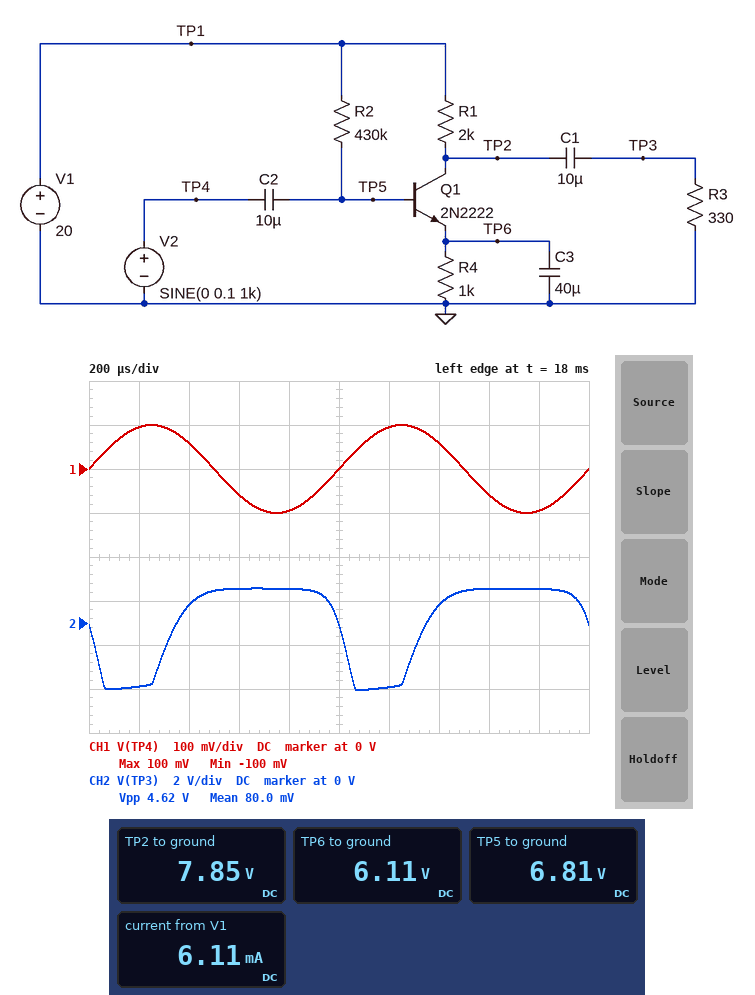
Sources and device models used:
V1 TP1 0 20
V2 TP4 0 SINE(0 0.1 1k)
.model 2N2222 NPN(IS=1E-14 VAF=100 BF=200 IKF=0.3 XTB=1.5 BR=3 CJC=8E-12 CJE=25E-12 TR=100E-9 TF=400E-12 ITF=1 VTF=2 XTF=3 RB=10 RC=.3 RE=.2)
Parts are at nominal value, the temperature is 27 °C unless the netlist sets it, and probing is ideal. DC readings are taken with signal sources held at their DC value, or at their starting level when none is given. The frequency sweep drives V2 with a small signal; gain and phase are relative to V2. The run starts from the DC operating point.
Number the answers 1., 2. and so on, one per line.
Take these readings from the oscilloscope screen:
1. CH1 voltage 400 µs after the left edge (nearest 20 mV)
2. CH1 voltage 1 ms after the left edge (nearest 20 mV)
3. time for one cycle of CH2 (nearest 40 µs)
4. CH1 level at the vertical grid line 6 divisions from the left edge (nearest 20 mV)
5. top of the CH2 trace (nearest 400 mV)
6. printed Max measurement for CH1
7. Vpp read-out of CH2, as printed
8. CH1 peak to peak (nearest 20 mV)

1. 60 mV
2. 0 V
3. 1.00 ms
4. 100 mV
5. 1.6 V
6. 100 mV
7. 4.62 V
8. 200 mV
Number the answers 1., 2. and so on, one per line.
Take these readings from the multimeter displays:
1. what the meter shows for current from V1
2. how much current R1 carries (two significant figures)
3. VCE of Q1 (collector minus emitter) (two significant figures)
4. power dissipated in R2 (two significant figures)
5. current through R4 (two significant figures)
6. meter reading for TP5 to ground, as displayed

1. 6.11 mA
2. 6.1 mA
3. 1.7 V
4. 400 µW
5. 6.1 mA
6. 6.81 V
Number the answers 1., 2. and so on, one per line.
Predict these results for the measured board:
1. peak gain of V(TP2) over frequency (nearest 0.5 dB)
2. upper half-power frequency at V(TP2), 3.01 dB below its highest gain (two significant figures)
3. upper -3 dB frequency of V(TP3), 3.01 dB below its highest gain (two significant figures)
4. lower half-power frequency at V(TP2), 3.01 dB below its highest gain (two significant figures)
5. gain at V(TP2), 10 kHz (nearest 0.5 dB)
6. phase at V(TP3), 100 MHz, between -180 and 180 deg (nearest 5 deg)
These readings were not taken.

1. 35.5 dB
2. 25 MHz
3. 25 MHz
4. 880 Hz
5. 35.5 dB
6. 90 deg
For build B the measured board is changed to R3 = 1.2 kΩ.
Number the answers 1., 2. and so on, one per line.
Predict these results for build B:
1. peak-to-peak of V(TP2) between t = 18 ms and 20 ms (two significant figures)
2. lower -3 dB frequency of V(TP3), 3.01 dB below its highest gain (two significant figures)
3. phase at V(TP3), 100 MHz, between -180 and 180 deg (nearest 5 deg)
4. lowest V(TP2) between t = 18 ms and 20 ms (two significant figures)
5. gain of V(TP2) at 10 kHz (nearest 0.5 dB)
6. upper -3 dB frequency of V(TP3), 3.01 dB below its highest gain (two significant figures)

1. 8.1 V
2. 860 Hz
3. 80 deg
4. 5.5 V
5. 44.0 dB
6. 11 MHz
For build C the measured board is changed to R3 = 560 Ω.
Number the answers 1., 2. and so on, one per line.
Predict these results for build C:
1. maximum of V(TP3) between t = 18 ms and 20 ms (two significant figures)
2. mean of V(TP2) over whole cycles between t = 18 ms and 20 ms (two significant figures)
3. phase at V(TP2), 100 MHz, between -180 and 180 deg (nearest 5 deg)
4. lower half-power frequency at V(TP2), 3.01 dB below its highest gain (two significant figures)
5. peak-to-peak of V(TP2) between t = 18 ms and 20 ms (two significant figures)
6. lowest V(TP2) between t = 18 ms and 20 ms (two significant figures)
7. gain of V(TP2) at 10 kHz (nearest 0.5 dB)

1. 2.3 V
2. 9.6 V
3. 85 deg
4. 870 Hz
5. 6.0 V
6. 5.7 V
7. 39.5 dB
